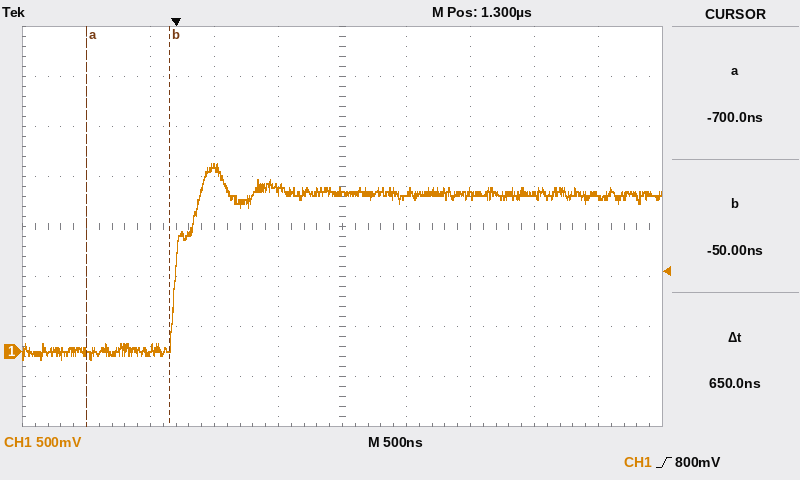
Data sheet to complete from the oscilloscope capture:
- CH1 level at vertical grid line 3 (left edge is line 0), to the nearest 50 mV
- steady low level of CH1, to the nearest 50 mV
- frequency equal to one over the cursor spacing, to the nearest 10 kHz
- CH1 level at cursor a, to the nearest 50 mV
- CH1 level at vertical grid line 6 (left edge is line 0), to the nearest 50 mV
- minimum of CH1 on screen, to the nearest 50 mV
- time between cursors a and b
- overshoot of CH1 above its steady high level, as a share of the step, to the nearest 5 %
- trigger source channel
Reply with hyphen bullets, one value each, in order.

- 1.85 V
- 0 mV
- 1.54 MHz
- 0 mV
- 1.55 V
- -100 mV
- 650 ns
- 20 %
- CH1
